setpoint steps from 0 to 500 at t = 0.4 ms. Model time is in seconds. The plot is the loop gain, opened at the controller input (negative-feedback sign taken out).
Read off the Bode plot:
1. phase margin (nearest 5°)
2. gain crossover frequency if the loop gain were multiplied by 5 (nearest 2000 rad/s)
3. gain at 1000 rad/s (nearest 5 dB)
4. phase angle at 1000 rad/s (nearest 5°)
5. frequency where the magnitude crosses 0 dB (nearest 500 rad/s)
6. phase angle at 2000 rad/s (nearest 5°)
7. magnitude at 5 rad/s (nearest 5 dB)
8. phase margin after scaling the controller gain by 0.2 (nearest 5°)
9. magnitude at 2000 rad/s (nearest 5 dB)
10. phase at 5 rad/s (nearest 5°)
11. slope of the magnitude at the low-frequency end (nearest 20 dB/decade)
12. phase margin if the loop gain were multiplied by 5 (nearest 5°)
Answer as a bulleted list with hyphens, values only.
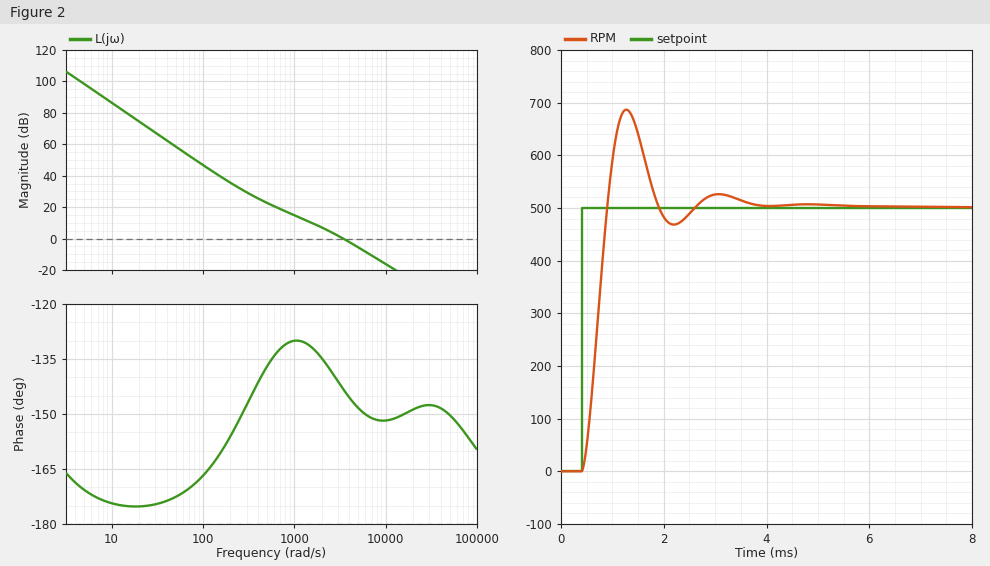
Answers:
- 35°
- 8000 rad/s
- 15 dB
- -130°
- 3500 rad/s
- -135°
- 100 dB
- 50°
- 5 dB
- -170°
- -40 dB/decade
- 30°
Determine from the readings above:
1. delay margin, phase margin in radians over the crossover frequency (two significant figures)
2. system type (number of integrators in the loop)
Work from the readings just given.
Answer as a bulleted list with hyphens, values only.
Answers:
- 0.00017 s
- 2
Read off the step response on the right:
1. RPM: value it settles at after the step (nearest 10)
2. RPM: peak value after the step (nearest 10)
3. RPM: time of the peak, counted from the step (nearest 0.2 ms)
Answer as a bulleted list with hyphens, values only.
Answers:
- 500
- 690
- 0.8 ms
